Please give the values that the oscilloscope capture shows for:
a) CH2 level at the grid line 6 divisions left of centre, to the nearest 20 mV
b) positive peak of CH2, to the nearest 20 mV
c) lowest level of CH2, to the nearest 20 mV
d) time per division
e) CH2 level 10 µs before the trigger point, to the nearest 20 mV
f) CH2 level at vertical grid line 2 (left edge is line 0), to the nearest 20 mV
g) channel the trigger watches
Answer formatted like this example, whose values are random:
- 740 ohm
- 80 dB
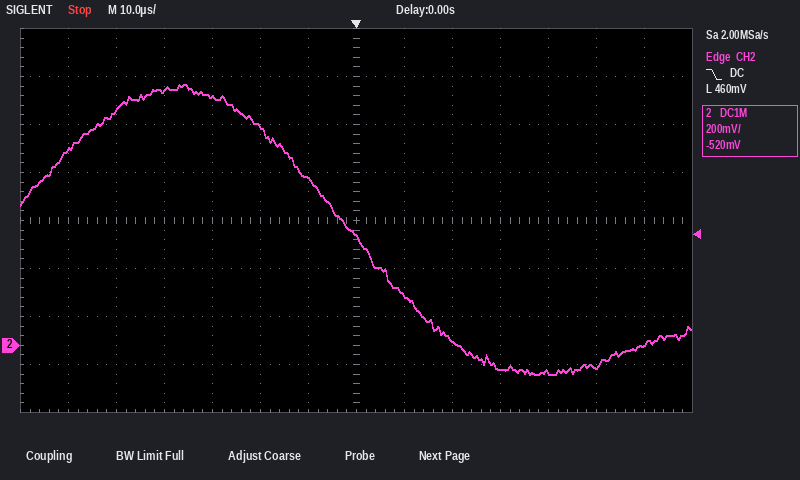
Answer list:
- 820 mV
- 1.08 V
- -120 mV
- 10 µs
- 700 mV
- 980 mV
- CH2
